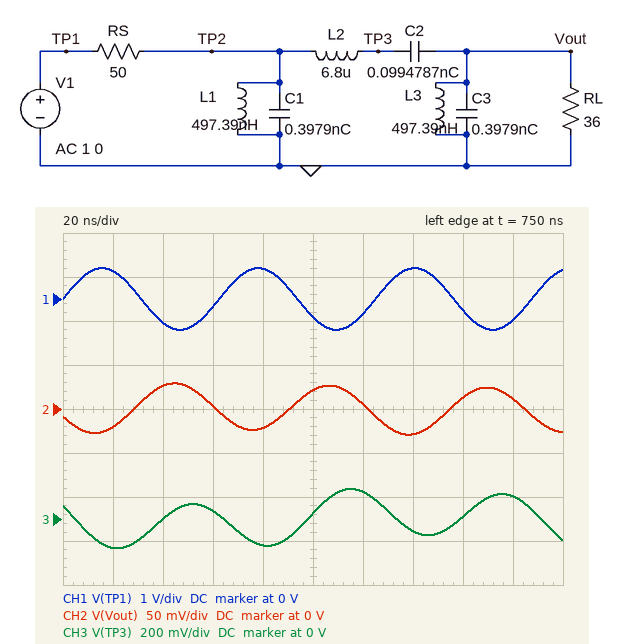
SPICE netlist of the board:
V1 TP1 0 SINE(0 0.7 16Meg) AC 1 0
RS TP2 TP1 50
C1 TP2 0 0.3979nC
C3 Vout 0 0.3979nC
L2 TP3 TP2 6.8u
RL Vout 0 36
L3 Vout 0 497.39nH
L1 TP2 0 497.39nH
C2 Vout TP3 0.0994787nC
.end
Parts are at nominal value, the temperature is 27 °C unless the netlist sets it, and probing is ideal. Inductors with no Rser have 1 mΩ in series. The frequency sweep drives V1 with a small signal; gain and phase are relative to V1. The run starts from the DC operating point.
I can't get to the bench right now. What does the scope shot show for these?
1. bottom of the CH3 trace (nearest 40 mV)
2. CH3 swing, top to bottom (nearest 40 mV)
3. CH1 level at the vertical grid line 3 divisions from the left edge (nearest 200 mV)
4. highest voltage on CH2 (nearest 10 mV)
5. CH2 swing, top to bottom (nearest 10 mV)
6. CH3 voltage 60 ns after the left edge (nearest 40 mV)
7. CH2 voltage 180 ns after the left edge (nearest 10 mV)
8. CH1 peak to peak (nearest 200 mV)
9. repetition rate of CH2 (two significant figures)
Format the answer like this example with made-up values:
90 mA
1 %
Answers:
-120 mV
280 mV
-200 mV
30 mV
60 mV
40 mV
10 mV
1.4 V
16 MHz
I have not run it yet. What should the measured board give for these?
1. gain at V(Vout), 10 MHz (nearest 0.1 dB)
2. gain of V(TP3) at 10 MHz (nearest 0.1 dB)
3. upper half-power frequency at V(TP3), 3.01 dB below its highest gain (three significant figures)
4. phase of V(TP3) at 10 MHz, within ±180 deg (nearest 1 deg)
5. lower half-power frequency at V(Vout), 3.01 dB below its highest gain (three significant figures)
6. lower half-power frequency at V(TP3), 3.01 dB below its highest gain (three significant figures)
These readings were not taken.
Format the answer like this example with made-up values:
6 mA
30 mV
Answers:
-19.2 dB
-6.3 dB
5.91 MHz
-133 deg
5.52 MHz
5.49 MHz
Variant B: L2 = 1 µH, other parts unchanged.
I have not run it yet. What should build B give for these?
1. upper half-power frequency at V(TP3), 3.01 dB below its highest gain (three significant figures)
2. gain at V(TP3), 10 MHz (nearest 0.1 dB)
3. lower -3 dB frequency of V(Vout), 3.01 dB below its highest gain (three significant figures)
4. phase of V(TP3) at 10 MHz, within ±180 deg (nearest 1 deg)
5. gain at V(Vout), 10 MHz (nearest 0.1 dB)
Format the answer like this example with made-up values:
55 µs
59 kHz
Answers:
21.5 MHz
2.7 dB
9.78 MHz
-15 deg
-10.2 dB
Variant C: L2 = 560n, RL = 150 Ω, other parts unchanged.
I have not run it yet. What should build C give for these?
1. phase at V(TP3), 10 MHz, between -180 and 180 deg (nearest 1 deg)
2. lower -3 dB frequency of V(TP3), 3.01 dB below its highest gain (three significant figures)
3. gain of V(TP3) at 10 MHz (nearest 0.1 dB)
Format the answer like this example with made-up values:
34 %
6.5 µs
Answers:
-14 deg
25.5 MHz
-1.2 dB
